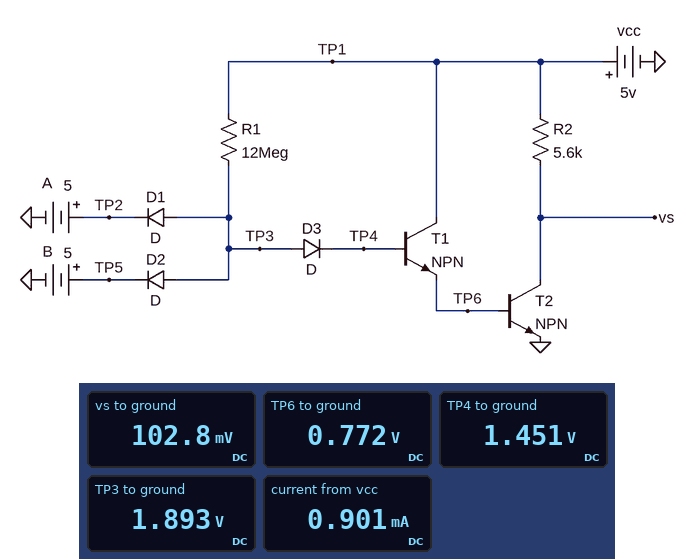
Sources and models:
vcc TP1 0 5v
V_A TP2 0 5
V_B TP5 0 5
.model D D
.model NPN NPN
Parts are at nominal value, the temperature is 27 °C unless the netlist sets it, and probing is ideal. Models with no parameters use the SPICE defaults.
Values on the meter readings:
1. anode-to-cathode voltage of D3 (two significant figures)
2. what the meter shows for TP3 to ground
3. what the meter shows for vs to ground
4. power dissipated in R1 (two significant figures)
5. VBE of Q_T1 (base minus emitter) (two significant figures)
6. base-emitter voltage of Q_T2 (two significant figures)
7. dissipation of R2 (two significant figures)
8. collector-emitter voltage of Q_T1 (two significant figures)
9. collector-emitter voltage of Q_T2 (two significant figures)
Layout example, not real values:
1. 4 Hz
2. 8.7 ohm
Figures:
1. 440 mV
2. 1.893 V
3. 102.8 mV
4. 800 nW
5. 680 mV
6. 770 mV
7. 4.3 mW
8. 4.2 V
9. 100 mV
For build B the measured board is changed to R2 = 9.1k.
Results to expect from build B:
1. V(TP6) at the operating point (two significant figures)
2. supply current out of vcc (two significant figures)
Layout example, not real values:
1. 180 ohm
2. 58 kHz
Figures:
1. 760 mV
2. 570 µA
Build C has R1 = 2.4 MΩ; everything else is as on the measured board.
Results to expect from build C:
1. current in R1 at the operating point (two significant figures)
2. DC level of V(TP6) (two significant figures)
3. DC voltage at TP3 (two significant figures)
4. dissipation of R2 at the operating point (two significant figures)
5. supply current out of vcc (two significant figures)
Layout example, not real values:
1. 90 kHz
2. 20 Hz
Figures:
1. 1.3 µA
2. 780 mV
3. 2.0 V
4. 4.4 mW
5. 1.0 mA
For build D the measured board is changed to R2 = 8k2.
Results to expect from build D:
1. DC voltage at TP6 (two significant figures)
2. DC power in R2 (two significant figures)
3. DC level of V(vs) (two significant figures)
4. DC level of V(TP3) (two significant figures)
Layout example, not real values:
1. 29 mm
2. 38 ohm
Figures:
1. 760 mV
2. 2.9 mW
3. 90 mV
4. 1.9 V
